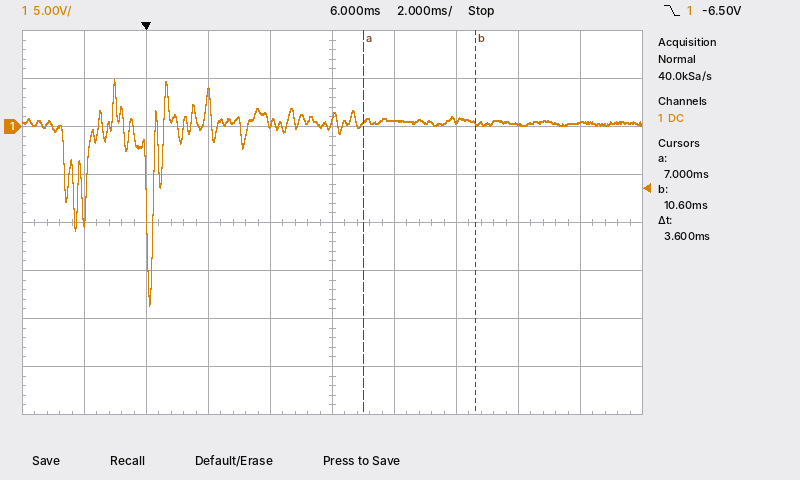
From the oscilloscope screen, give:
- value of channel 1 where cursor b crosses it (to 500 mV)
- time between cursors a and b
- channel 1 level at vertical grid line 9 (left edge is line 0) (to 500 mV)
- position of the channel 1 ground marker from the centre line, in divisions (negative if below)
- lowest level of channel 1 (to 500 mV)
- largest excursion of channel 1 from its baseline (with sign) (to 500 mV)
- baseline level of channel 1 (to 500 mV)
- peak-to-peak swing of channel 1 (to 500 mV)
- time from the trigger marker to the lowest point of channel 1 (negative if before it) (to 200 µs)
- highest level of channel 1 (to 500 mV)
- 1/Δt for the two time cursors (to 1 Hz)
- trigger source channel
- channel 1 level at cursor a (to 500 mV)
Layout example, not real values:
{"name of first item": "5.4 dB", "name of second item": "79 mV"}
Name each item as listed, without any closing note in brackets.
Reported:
{"value of channel 1 where cursor b crosses it": "500 mV", "time between cursors a and b": "3.6 ms", "channel 1 level at vertical grid line 9 (left edge is line 0)": "500 mV", "position of the channel 1 ground marker from the centre line, in divisions": "+2.0 div", "lowest level of channel 1": "-18.5 V", "largest excursion of channel 1 from its baseline (with sign)": "-19.0 V", "baseline level of channel 1": "500 mV", "peak-to-peak swing of channel 1": "23.5 V", "time from the trigger marker to the lowest point of channel 1 (negative if before it)": "+200 µs", "highest level of channel 1": "5.0 V", "1/Δt for the two time cursors": "278 Hz", "trigger source channel": "channel 1", "channel 1 level at cursor a": "500 mV"}
